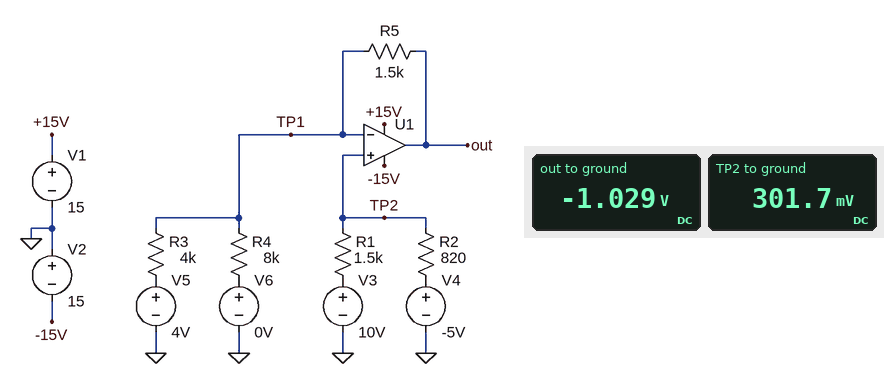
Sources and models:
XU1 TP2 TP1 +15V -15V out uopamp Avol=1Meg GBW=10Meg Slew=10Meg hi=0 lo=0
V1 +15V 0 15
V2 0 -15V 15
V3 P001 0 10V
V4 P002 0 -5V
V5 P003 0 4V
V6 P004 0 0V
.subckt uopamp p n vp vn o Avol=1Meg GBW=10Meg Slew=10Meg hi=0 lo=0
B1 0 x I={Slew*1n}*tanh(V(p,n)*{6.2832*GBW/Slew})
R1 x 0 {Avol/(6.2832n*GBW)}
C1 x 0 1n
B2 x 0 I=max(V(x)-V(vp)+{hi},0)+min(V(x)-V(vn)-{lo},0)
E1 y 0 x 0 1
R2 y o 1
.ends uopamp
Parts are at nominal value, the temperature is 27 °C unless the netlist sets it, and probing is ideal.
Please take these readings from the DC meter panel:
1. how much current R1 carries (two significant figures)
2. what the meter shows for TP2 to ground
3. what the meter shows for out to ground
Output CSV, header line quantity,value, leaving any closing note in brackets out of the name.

quantity,value
how much current R1 carries,6.5 mA
what the meter shows for TP2 to ground,301.7 mV
what the meter shows for out to ground,-1.029 V
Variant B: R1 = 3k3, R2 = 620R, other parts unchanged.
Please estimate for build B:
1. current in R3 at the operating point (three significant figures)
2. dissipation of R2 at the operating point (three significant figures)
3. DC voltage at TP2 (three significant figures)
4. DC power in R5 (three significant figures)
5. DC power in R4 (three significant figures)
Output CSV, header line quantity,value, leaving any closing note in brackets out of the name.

quantity,value
current in R3 at the operating point,1.66 mA
dissipation of R2 at the operating point,9.08 mW
DC voltage at TP2,-2.63 V
DC power in R5,5.91 mW
DC power in R4,863 µW
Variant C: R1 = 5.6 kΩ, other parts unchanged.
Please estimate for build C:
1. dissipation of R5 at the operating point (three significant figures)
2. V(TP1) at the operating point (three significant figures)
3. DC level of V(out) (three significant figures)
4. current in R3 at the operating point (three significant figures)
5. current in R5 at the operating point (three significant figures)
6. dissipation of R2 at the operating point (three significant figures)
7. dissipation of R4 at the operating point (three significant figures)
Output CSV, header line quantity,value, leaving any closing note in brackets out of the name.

quantity,value
dissipation of R5 at the operating point,6.98 mW
V(TP1) at the operating point,-3.08 V
DC level of V(out),-6.32 V
current in R3 at the operating point,1.77 mA
current in R5 at the operating point,2.16 mA
dissipation of R2 at the operating point,4.48 mW
dissipation of R4 at the operating point,1.19 mW
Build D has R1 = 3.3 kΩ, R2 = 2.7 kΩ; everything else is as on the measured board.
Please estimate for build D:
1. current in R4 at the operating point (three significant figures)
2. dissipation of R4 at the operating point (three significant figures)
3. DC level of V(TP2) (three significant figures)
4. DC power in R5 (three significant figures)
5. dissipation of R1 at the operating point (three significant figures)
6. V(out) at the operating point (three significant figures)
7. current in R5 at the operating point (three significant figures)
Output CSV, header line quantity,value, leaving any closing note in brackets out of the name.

quantity,value
current in R4 at the operating point,219 µA
dissipation of R4 at the operating point,383 µW
DC level of V(TP2),1.75 V
DC power in R5,177 µW
dissipation of R1 at the operating point,20.6 mW
V(out) at the operating point,1.23 V
current in R5 at the operating point,344 µA
